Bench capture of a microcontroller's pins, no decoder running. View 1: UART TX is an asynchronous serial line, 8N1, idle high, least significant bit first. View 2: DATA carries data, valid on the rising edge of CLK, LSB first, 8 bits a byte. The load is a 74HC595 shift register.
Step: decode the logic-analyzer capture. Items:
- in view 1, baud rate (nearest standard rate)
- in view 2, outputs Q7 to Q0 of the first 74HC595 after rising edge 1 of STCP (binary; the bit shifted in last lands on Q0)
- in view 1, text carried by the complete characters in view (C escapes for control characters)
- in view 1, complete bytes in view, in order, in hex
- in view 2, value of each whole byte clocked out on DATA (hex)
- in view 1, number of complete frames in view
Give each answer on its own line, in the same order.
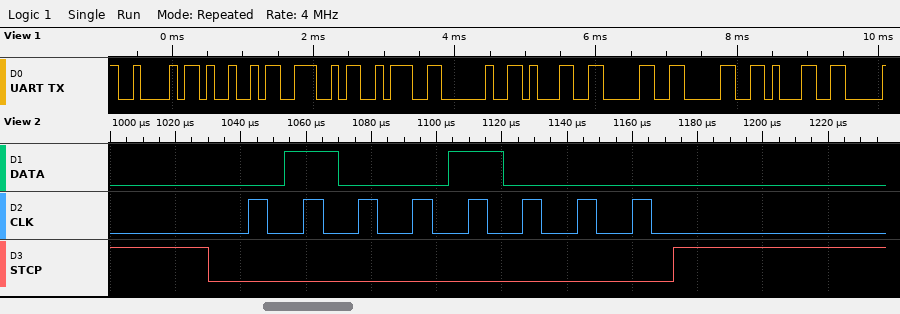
9600 baud
01001000
"BIN: 1001"
42 49 4E 3A 20 31 30 30 31
12
9
